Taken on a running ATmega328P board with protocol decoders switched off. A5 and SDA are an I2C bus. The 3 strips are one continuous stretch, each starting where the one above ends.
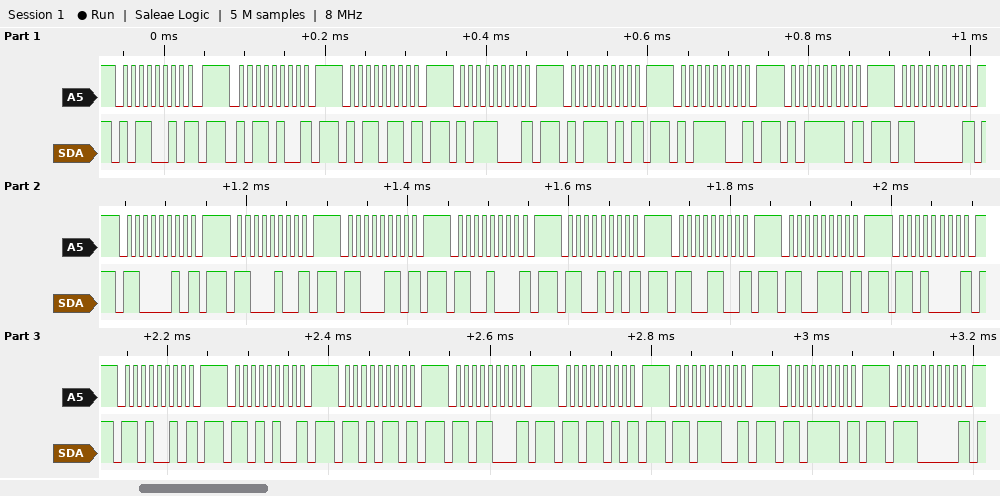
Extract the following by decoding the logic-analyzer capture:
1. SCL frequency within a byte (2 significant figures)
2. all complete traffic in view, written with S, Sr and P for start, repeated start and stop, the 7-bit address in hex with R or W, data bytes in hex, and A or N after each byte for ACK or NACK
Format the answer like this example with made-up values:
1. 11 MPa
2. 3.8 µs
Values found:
1. 100 kHz
2. S 59W N P S 5AW N P S 5BW N P S 5CW N P S 5DW N P S 5EW N P S 5FW N P S 60W N P S 61W N P S 62W N P S 63W N P S 64W N P S 65W N P S 66W N P S 67W N P S 68W N P S 69W N P S 6AW N P S 6BW N P S 6CW N P S 6DW N P S 6EW N P S 6FW N P S 70W N P
